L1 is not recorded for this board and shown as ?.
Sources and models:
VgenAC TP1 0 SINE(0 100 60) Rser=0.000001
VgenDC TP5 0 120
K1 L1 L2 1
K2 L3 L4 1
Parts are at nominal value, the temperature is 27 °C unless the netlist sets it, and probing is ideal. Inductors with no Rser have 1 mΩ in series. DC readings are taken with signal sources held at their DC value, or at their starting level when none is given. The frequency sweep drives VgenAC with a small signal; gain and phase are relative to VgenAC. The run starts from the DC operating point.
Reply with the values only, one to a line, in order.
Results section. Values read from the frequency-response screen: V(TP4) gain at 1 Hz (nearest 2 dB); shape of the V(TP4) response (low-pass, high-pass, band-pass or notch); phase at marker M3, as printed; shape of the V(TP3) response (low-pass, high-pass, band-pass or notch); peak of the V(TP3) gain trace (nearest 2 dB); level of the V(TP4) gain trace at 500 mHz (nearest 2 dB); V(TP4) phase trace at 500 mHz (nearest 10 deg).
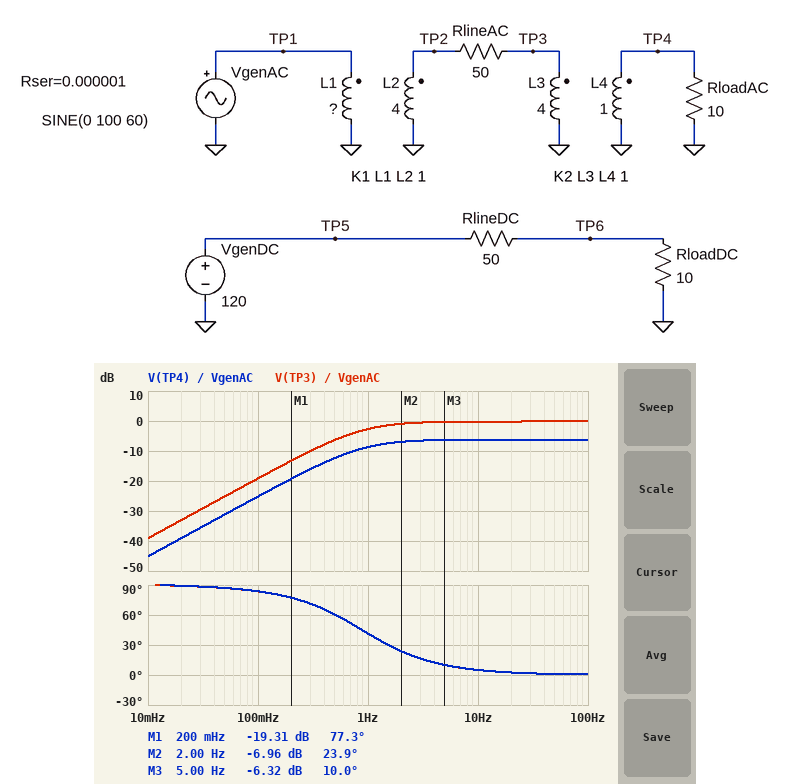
-8 dB
high-pass
10.0 deg
high-pass
0 dB
-12 dB
60 deg
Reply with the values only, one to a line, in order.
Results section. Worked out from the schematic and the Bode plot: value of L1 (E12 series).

820 mH
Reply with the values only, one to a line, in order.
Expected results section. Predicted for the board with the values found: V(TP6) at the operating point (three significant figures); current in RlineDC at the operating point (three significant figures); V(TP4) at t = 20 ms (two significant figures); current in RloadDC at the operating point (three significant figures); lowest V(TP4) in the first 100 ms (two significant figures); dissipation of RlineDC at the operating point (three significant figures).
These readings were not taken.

20.0 V
2.00 A
46 V
2.00 A
-50 V
200 W
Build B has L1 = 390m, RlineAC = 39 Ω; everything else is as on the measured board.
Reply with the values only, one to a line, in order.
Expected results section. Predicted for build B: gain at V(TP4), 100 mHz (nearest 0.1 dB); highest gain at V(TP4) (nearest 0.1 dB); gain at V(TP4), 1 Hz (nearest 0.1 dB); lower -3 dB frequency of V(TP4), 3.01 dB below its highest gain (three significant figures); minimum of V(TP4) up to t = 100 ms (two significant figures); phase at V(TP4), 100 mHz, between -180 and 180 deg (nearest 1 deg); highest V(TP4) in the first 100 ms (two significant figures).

-19.8 dB
-1.8 dB
-3.9 dB
786 mHz
-82 V
83 deg
80 V
